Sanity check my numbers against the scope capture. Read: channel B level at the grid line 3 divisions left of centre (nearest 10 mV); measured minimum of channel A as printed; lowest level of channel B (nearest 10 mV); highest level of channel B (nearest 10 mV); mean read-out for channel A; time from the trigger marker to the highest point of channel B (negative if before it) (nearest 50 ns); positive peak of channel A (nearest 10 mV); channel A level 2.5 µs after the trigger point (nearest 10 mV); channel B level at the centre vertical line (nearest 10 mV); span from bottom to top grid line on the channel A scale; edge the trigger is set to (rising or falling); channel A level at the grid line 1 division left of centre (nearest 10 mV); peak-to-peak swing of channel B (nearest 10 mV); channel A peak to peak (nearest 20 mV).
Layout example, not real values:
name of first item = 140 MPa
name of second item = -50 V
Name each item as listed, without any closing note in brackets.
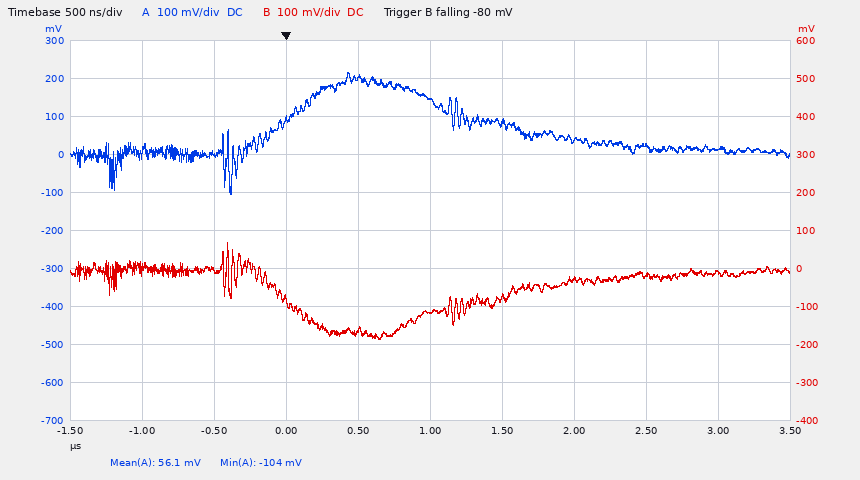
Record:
channel B level at the grid line 3 divisions left of centre = 0 mV
measured minimum of channel A as printed = -104 mV
lowest level of channel B = -190 mV
highest level of channel B = 70 mV
mean read-out for channel A = 56.1 mV
time from the trigger marker to the highest point of channel B (negative if before it) = -400 ns
positive peak of channel A = 220 mV
channel A level 2.5 µs after the trigger point = 20 mV
channel B level at the centre vertical line = -110 mV
span from bottom to top grid line on the channel A scale = 1 V
edge the trigger is set to = falling
channel A level at the grid line 1 division left of centre = 200 mV
peak-to-peak swing of channel B = 260 mV
channel A peak to peak = 320 mV
